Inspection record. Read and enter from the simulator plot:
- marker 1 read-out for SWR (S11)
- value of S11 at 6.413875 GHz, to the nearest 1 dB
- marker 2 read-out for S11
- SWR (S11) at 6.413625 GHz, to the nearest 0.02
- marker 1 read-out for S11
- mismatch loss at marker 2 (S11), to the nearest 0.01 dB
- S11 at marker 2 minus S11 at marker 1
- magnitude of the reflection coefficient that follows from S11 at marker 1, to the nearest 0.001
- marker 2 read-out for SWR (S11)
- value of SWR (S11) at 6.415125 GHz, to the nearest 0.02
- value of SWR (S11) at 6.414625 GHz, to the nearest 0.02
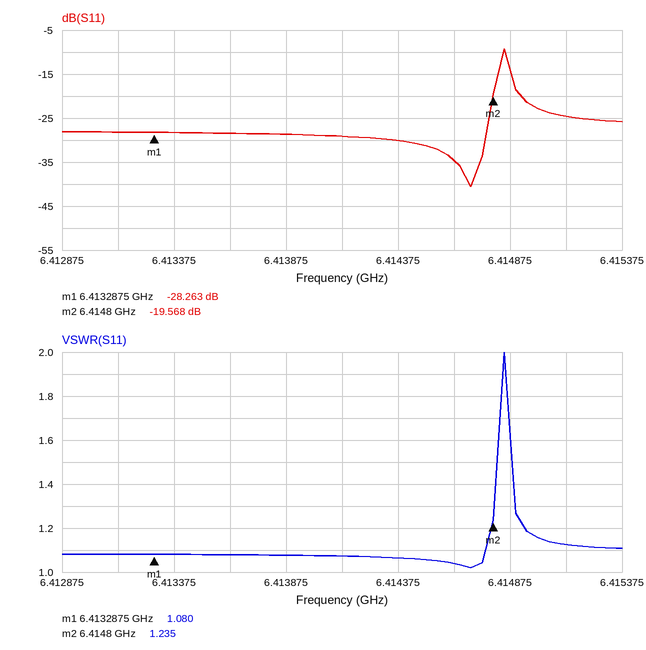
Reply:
1.080
-29 dB
-19.568 dB
1.08
-28.263 dB
0.05 dB
8.695 dB
0.039
1.235
1.12
1.04
